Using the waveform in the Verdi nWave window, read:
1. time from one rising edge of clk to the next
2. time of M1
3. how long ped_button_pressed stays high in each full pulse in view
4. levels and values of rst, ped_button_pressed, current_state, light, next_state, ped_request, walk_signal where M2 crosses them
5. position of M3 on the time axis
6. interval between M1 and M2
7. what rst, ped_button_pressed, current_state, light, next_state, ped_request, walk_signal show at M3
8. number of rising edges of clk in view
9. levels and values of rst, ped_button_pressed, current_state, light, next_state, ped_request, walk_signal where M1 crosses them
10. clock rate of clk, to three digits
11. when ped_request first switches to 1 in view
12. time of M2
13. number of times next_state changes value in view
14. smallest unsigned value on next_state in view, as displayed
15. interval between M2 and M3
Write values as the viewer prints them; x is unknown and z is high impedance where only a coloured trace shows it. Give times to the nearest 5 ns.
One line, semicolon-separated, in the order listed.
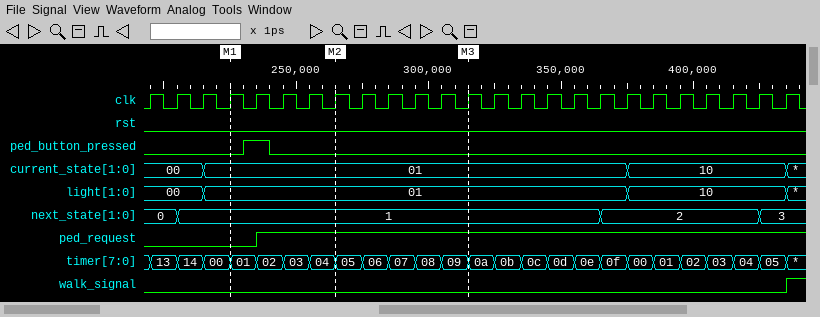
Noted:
10 ns; 225 ns; 10 ns; rst=0, ped_button_pressed=0, current_state=01, light=01, next_state=1, ped_request=1, walk_signal=0; 315 ns; 40 ns; rst=0, ped_button_pressed=0, current_state=01, light=01, next_state=1, ped_request=1, walk_signal=0; 25; rst=0, ped_button_pressed=0, current_state=01, light=01, next_state=1, ped_request=0, walk_signal=0; 100 MHz; 235 ns; 265 ns; 3; 0; 50 ns
